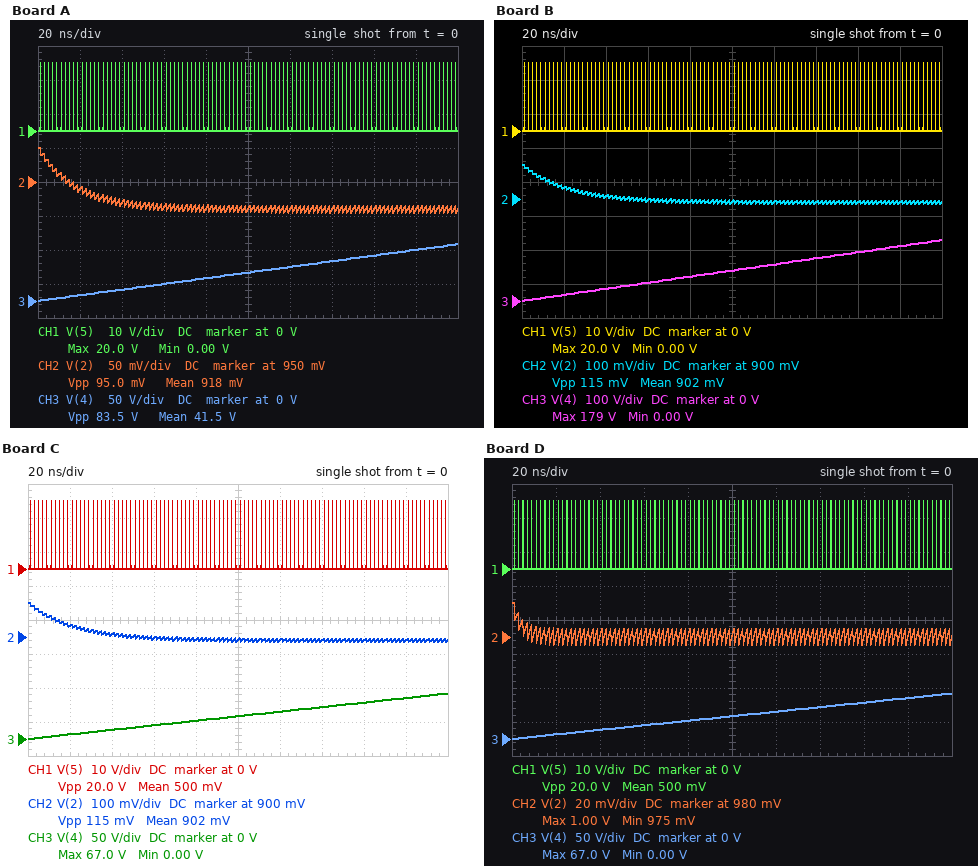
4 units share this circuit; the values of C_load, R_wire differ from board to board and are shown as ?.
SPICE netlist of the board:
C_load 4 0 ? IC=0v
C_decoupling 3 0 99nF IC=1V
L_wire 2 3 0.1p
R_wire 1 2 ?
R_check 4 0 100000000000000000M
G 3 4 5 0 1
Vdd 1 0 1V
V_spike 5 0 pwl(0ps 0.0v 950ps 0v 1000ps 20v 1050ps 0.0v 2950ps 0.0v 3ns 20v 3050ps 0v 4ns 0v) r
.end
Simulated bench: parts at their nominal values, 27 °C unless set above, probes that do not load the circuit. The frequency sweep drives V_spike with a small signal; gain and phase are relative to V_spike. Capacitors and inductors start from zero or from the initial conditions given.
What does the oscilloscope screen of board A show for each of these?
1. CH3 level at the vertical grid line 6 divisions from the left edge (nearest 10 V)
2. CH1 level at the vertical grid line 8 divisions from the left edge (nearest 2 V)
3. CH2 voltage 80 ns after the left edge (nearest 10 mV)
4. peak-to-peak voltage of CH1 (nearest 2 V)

50 V
0 V
910 mV
20 V
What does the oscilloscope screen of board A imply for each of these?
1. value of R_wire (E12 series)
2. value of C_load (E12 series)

0.18 Ω
1.2 nF
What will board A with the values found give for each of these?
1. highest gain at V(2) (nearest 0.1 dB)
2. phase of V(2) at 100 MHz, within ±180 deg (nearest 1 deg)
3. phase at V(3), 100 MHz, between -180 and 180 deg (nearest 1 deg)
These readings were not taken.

-14.9 dB
95 deg
95 deg
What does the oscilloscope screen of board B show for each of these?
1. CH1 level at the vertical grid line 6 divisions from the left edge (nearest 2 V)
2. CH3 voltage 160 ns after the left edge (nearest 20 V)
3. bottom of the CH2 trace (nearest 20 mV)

0 V
140 V
880 mV
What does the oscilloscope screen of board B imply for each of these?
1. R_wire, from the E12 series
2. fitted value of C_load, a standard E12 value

0.22 Ω
560 pF
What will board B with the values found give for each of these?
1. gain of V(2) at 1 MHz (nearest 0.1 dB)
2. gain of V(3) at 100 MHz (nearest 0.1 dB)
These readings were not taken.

-13.2 dB
-35.9 dB
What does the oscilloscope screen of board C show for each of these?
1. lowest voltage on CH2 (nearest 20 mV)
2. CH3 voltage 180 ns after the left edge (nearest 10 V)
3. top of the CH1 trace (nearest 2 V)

880 mV
60 V
20 V
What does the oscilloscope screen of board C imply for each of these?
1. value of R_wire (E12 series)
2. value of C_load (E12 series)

0.22 Ω
1.5 nF
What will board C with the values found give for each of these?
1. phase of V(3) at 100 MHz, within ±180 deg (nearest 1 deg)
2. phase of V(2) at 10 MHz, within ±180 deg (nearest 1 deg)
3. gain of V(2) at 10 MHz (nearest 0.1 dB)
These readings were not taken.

94 deg
126 deg
-17.7 dB
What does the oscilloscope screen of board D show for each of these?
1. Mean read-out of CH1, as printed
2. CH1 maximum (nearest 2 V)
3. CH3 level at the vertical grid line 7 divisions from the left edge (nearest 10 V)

500 mV
20 V
50 V
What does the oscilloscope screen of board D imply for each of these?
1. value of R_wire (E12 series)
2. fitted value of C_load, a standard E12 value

0.039 Ω
1.5 nF
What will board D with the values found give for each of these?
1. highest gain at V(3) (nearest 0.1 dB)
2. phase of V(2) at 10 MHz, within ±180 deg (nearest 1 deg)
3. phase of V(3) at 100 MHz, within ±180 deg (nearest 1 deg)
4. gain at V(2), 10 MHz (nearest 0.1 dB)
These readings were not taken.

-28.2 dB
166 deg
112 deg
-28.4 dB
